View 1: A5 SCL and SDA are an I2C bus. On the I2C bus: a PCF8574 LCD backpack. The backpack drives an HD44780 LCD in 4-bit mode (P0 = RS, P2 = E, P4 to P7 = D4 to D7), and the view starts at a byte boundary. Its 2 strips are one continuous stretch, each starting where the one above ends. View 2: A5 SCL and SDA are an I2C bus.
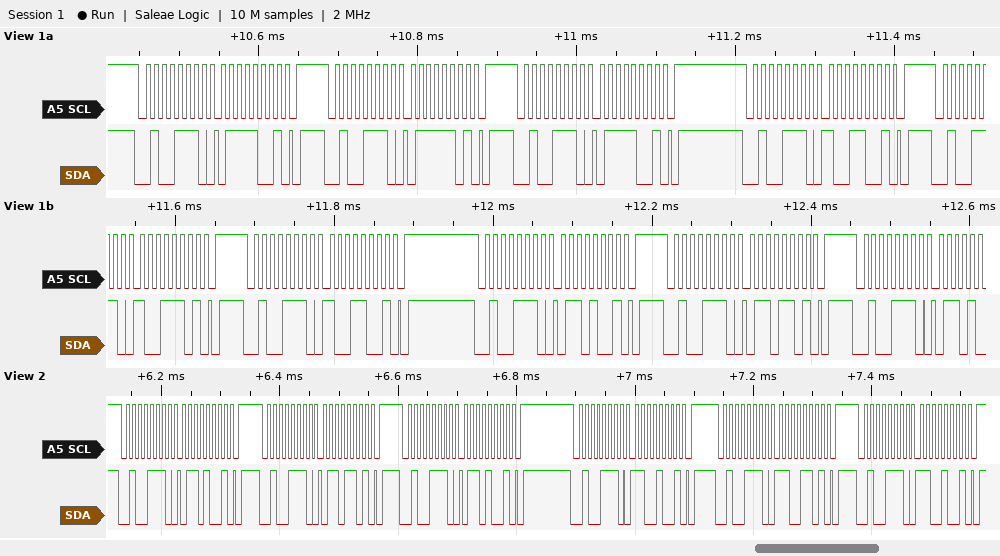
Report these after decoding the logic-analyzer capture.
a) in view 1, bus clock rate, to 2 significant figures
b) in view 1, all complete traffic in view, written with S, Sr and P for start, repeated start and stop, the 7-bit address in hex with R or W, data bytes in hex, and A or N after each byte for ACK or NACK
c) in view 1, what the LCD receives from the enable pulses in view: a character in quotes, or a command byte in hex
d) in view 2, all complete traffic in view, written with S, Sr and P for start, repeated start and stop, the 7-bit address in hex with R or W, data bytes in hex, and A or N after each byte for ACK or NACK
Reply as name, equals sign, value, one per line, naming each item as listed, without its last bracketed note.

in view 1, bus clock rate, to 2 significant figures = 100 kHz
in view 1, all complete traffic in view, written with S, Sr and P for start, repeated start and stop, the 7-bit address in hex with R or W, data bytes in hex, and A or N after each byte for ACK or NACK = S 27W A 79 A P S 27W A 7D A P S 27W A 79 A P S 27W A 99 A P S 27W A 9D A P S 27W A 99 A P S 27W A 69 A P S 27W A 6D A P S 27W A
in view 1, what the LCD receives from the enable pulses in view: a character in quotes, or a command byte in hex = 'y'
in view 2, all complete traffic in view, written with S, Sr and P for start, repeated start and stop, the 7-bit address in hex with R or W, data bytes in hex, and A or N after each byte for ACK or NACK = S 27W A 69 A P S 27W A 6D A P S 27W A 69 A P S 27W A C9 A P S 27W A CD A P S 27W A C9 A P
